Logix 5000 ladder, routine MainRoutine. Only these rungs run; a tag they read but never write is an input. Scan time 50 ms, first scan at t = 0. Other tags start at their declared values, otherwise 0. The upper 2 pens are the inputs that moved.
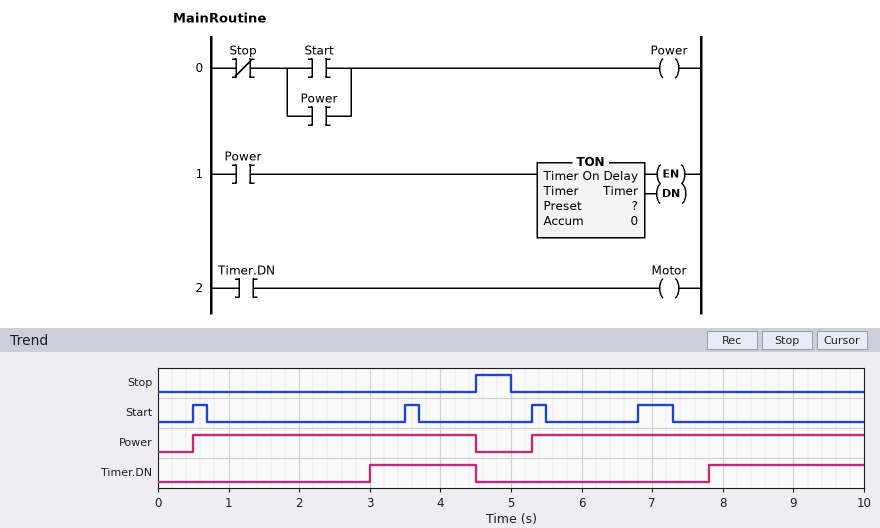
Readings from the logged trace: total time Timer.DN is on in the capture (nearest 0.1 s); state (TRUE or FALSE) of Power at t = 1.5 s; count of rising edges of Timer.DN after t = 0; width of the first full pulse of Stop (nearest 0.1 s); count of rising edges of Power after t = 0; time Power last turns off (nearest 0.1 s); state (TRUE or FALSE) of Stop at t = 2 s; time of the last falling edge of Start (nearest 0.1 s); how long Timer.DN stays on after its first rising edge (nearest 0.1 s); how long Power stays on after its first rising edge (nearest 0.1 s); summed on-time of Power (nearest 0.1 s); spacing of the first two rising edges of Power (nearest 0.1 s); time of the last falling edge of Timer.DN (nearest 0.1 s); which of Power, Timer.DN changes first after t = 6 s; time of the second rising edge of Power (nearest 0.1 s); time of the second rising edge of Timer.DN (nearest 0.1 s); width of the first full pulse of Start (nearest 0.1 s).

3.7 s
TRUE
2
0.5 s
2
4.5 s
FALSE
7.3 s
1.5 s
4.0 s
8.7 s
4.8 s
4.5 s
Timer.DN
5.3 s
7.8 s
0.2 s
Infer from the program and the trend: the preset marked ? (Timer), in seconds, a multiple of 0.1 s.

2.5 s
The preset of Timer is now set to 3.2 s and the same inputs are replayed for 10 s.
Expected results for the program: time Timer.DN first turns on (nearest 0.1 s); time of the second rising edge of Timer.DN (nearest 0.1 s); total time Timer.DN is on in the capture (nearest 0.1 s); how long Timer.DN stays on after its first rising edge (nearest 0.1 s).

3.7 s
8.5 s
2.3 s
0.8 s
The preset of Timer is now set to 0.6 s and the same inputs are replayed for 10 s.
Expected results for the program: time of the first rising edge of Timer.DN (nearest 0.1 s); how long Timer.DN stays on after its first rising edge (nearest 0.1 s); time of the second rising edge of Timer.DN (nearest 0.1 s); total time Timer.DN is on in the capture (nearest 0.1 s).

1.1 s
3.4 s
5.9 s
7.5 s
